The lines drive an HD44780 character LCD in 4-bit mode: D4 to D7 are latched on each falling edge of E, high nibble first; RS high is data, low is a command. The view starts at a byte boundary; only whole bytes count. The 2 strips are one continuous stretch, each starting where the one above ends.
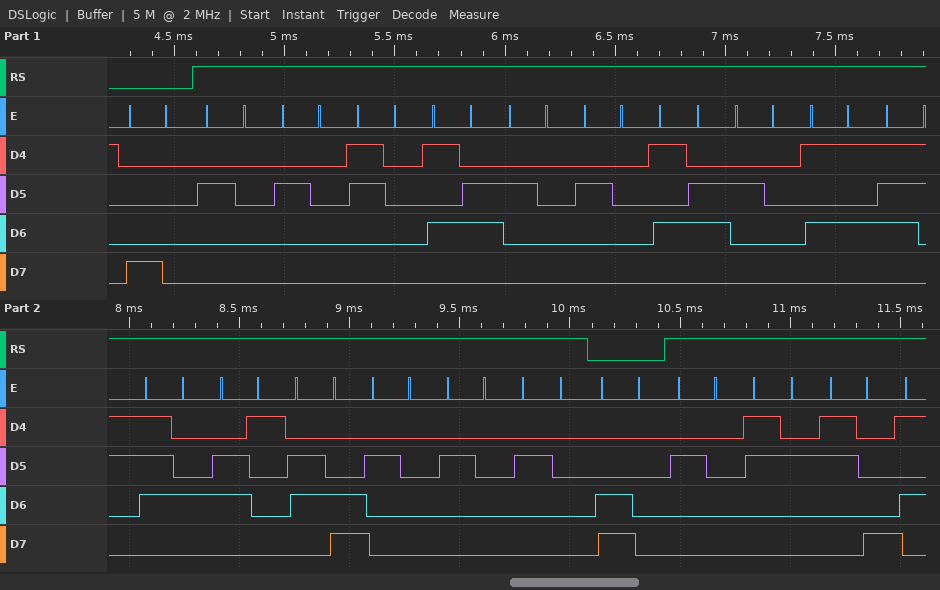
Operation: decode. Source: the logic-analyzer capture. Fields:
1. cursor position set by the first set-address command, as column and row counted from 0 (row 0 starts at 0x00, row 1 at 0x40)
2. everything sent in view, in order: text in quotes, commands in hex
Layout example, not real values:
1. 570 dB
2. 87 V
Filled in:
1. column 0, row 0
2. 0x80 "  0V  V Ustal   " 0xC0 " 28"
